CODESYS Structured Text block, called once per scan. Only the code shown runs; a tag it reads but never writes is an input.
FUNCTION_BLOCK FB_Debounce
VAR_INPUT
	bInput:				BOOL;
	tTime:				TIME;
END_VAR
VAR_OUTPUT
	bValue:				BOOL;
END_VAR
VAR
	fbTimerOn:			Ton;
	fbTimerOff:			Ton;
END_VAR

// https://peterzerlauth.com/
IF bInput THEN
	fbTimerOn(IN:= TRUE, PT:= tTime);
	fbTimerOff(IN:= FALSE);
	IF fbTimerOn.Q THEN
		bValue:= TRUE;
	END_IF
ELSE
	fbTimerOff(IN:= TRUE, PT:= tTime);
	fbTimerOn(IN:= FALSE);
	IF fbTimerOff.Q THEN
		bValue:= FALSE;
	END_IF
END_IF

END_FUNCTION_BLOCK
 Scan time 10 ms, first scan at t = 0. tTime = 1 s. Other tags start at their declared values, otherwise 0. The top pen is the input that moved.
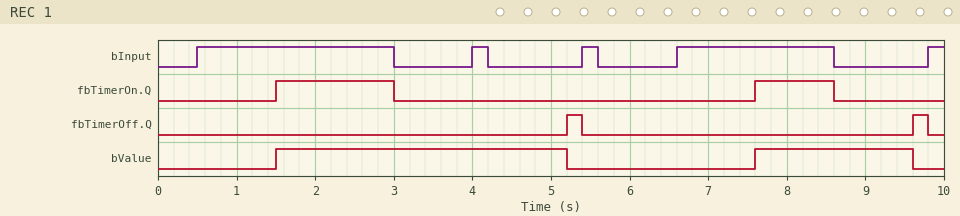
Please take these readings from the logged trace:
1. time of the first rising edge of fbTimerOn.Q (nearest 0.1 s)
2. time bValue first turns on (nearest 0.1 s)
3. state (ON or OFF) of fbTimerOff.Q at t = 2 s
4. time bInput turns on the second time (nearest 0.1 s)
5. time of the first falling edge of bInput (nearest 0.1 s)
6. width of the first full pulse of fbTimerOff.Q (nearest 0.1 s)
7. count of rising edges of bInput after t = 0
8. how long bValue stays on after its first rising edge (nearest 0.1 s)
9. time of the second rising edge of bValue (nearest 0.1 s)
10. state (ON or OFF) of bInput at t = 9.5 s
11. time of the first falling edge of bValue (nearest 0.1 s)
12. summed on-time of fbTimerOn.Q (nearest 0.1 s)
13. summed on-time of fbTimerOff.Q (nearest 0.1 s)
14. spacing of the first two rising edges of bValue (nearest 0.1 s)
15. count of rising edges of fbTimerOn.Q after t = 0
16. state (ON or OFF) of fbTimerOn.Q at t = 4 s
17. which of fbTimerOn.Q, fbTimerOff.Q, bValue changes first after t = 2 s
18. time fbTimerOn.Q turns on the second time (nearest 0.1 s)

1.5 s
1.5 s
OFF
4.0 s
3.0 s
0.2 s
5
3.7 s
7.6 s
OFF
5.2 s
2.5 s
0.4 s
6.1 s
2
OFF
fbTimerOn.Q
7.6 s
